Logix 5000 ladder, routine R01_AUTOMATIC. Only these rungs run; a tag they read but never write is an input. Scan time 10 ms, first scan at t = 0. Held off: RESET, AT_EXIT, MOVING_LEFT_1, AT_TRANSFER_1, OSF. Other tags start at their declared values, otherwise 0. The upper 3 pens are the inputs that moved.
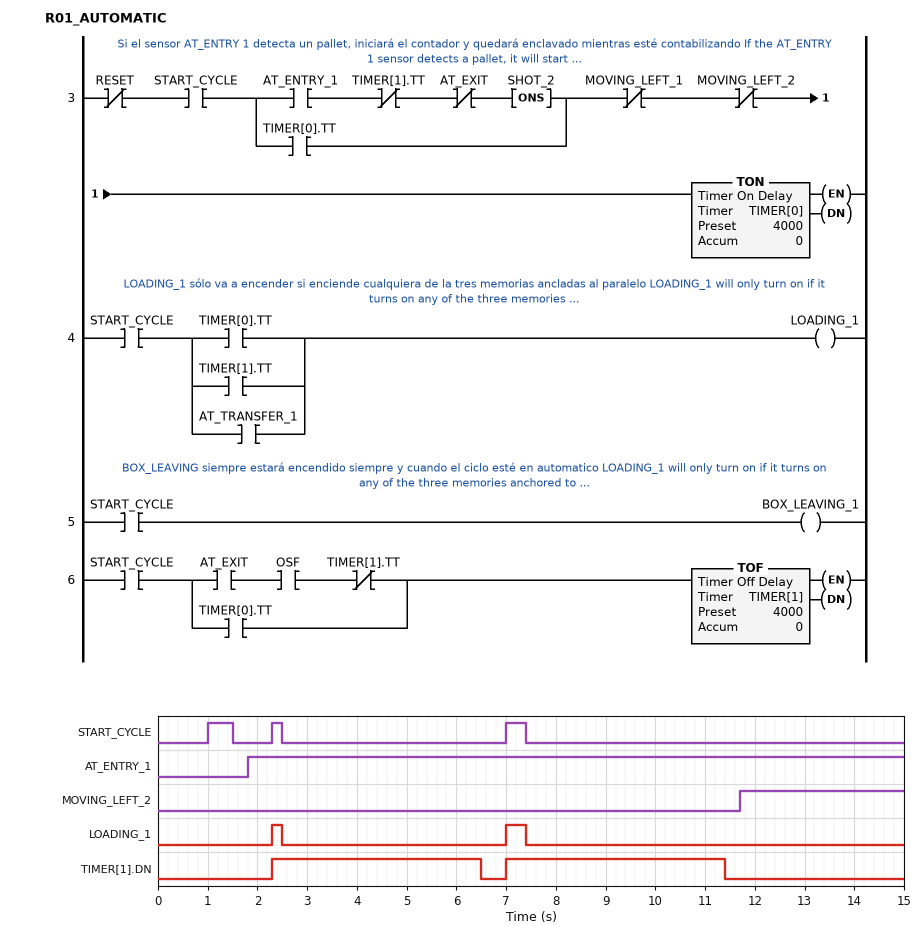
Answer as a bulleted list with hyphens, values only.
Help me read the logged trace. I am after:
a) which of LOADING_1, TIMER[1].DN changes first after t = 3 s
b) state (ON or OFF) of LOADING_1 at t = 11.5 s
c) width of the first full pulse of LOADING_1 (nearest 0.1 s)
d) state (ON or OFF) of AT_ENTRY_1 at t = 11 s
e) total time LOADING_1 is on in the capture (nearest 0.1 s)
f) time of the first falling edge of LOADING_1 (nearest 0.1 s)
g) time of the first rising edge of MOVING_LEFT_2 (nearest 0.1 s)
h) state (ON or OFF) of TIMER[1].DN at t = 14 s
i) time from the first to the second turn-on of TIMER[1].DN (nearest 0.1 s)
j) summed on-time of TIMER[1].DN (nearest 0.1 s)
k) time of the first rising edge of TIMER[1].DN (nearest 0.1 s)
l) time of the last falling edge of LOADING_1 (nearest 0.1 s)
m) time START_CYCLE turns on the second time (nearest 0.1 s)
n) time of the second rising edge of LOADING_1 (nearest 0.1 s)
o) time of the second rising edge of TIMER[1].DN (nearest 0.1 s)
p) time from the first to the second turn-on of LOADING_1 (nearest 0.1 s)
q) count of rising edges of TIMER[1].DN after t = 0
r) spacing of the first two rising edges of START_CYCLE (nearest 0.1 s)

- TIMER[1].DN
- OFF
- 0.2 s
- ON
- 0.6 s
- 2.5 s
- 11.7 s
- OFF
- 4.7 s
- 8.6 s
- 2.3 s
- 7.4 s
- 2.3 s
- 7.0 s
- 7.0 s
- 4.7 s
- 2
- 1.3 s
